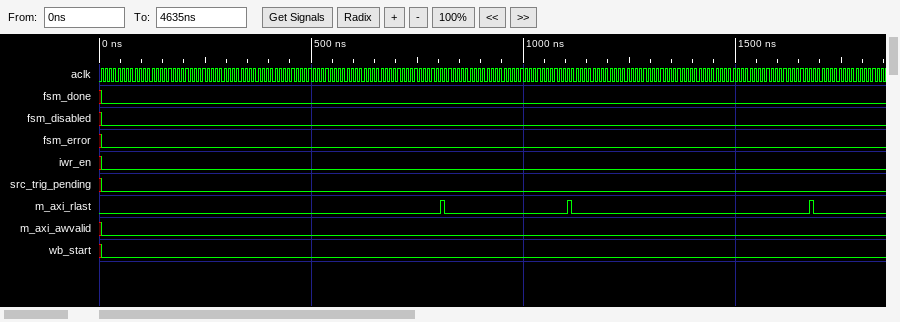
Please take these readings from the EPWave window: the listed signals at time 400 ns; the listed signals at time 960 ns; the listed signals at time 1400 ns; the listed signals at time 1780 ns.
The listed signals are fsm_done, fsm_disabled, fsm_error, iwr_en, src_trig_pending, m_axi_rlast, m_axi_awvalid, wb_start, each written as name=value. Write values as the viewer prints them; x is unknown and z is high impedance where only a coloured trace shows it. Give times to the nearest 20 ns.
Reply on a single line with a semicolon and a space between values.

fsm_done=0, fsm_disabled=0, fsm_error=0, iwr_en=0, src_trig_pending=0, m_axi_rlast=0, m_axi_awvalid=0, wb_start=0; fsm_done=0, fsm_disabled=0, fsm_error=0, iwr_en=0, src_trig_pending=0, m_axi_rlast=0, m_axi_awvalid=0, wb_start=0; fsm_done=0, fsm_disabled=0, fsm_error=0, iwr_en=0, src_trig_pending=0, m_axi_rlast=0, m_axi_awvalid=0, wb_start=0; fsm_done=0, fsm_disabled=0, fsm_error=0, iwr_en=0, src_trig_pending=0, m_axi_rlast=0, m_axi_awvalid=0, wb_start=0
